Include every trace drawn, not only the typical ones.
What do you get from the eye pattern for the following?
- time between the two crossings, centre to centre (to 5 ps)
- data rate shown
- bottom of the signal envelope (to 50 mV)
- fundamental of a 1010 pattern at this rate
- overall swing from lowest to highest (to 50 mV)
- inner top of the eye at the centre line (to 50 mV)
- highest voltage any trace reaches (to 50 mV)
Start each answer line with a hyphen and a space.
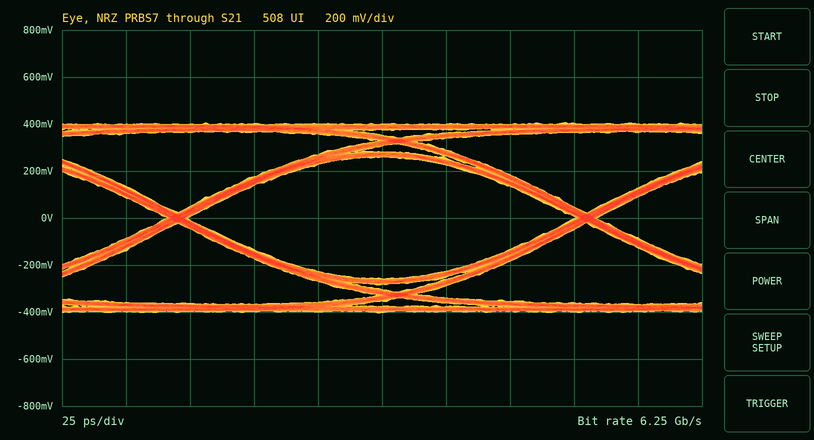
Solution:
- 160 ps
- 6.25 Gb/s
- -400 mV
- 3.125 GHz
- 800 mV
- 250 mV
- 400 mV
